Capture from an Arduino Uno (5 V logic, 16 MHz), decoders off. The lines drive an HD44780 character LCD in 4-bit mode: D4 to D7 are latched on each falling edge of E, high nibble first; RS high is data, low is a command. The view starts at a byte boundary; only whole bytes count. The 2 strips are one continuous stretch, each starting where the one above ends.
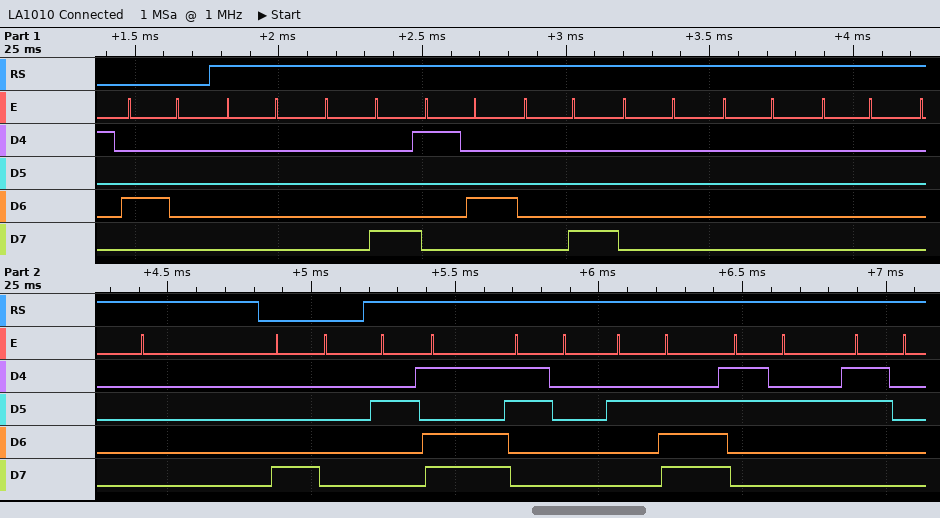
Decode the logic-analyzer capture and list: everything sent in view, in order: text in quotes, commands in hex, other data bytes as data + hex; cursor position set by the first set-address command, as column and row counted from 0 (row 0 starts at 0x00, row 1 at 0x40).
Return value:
0x40 data 00 08 14 08 00 00 00 00 0x80 "-0.20"
column 0, row 0
